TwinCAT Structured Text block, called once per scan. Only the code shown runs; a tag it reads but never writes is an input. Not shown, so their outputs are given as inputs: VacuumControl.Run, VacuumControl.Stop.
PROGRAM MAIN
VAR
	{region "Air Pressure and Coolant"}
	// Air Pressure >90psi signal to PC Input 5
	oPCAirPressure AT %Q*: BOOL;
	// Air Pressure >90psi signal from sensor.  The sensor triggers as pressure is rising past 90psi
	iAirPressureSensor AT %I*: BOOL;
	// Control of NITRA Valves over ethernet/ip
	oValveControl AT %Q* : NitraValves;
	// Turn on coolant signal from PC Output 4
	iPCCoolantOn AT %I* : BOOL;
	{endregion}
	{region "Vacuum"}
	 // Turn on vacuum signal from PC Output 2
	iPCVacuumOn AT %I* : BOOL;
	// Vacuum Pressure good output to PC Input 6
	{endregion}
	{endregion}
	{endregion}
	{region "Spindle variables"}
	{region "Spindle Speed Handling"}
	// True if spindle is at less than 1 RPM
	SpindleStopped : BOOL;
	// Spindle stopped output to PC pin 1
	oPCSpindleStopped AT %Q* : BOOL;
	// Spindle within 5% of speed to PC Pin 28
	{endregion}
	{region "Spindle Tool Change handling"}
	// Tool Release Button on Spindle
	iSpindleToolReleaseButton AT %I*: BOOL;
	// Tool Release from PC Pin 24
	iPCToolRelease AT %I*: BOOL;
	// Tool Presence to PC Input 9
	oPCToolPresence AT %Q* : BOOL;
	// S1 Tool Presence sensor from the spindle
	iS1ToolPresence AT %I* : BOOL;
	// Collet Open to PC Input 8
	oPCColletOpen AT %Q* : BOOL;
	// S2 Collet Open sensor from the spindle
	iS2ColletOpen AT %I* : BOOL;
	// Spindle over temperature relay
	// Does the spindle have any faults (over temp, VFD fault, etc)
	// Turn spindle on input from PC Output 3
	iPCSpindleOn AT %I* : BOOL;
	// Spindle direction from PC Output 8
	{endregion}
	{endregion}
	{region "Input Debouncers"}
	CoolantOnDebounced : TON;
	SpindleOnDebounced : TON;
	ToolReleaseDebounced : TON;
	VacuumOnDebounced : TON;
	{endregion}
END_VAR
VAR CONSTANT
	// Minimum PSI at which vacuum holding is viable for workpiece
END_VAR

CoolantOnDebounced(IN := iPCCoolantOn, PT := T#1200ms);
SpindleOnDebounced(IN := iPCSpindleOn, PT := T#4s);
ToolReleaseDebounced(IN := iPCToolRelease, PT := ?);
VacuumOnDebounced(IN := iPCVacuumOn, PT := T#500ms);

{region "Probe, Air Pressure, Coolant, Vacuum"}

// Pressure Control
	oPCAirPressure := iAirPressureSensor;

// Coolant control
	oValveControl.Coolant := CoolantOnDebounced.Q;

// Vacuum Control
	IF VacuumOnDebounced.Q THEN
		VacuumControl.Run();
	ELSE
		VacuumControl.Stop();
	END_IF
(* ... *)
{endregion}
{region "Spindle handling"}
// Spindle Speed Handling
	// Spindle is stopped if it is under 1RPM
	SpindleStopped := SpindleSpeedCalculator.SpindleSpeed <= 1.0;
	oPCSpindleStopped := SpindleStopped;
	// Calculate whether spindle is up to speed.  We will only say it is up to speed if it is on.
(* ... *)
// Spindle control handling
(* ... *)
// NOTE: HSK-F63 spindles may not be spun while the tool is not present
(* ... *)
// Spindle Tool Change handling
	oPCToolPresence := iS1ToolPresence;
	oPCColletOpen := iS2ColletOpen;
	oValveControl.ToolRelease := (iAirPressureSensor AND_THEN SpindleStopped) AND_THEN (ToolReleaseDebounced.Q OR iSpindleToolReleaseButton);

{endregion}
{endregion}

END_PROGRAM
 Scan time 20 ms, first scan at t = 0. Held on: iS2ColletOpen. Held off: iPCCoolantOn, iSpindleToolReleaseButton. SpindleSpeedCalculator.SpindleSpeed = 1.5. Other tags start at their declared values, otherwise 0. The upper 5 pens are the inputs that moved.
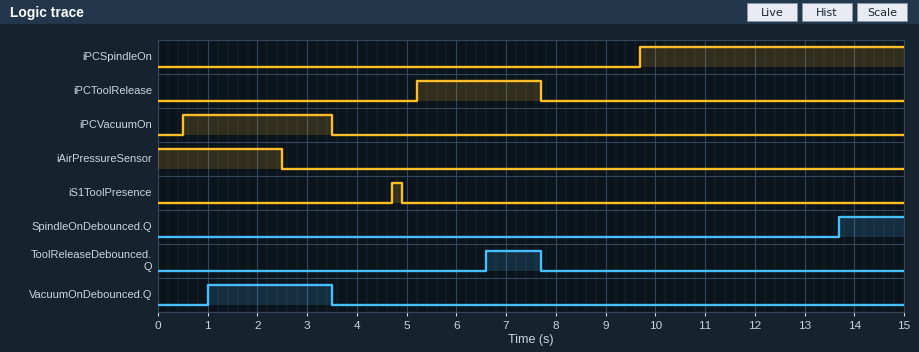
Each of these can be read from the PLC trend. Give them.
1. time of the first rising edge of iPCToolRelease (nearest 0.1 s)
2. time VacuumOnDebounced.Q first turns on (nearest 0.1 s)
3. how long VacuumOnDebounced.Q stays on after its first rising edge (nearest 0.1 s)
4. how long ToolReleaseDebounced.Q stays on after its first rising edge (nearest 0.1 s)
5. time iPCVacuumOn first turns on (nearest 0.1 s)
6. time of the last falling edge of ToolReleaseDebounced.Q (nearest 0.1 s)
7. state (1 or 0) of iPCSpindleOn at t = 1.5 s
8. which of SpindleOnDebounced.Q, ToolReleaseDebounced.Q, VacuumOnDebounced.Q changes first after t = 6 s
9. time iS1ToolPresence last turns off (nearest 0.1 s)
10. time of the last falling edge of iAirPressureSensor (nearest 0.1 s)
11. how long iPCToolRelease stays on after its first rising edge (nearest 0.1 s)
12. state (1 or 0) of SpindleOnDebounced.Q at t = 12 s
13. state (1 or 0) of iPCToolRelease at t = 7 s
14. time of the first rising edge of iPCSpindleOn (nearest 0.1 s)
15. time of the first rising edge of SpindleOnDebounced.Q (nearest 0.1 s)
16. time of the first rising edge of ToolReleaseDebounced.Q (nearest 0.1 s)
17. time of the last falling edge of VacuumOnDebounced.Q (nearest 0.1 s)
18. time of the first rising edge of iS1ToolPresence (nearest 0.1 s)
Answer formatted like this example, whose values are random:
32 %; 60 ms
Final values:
5.2 s; 1.0 s; 2.5 s; 1.1 s; 0.5 s; 7.7 s; 0; ToolReleaseDebounced.Q; 4.9 s; 2.5 s; 2.5 s; 0; 1; 9.7 s; 13.7 s; 6.6 s; 3.5 s; 4.7 s
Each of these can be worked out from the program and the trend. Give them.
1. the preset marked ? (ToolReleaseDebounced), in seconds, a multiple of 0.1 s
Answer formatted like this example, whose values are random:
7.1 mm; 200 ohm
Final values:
1.4 s
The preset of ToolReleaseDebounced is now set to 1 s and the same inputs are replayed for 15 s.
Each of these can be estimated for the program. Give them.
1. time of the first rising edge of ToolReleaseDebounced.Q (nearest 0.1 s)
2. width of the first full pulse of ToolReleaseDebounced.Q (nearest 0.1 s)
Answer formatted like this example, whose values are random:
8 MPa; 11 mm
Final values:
6.2 s; 1.5 s
